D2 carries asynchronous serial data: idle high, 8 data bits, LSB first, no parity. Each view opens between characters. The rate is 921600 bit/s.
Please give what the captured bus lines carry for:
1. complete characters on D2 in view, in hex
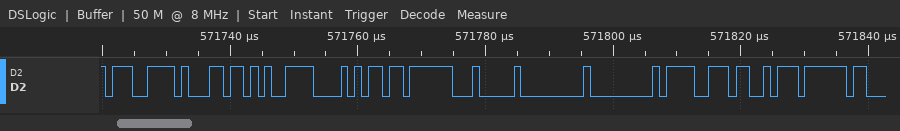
E7, B1, E5, A8, FB, 04, 00, 00, CF, D3, BF
